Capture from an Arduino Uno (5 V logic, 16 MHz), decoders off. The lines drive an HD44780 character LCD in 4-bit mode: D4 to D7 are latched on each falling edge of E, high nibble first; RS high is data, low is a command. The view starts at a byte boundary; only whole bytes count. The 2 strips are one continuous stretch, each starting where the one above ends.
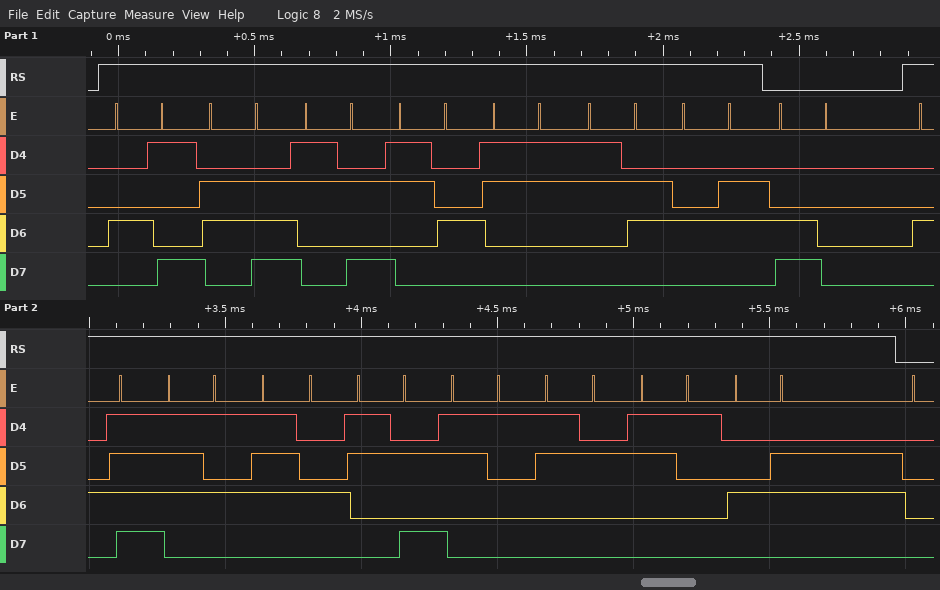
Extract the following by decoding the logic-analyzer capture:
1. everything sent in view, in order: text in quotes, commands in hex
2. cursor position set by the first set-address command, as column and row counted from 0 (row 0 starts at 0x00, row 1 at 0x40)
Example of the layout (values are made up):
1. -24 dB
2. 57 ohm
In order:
1. "In:436F" 0xC0 "Out:121F"
2. column 0, row 1
